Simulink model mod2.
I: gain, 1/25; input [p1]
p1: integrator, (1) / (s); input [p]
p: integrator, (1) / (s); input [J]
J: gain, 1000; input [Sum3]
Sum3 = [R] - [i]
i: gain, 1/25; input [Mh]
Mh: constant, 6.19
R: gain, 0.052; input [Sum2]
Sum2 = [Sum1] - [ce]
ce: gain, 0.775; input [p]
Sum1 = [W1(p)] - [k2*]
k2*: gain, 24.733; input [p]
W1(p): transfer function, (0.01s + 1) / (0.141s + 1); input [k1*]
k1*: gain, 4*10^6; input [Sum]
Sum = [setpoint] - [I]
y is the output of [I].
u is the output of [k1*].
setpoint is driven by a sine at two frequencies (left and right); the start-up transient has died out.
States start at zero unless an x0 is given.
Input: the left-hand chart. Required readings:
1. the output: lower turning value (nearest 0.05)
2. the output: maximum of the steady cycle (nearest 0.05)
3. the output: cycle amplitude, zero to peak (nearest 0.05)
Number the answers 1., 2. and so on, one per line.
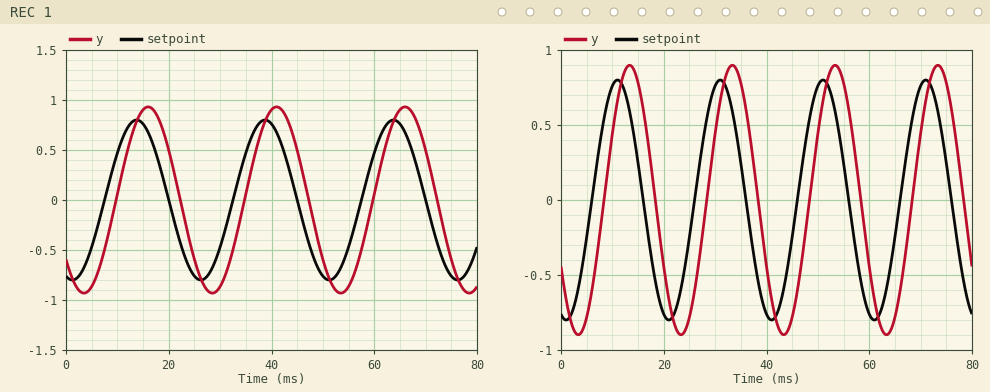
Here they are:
1. -0.95
2. 0.95
3. 0.95
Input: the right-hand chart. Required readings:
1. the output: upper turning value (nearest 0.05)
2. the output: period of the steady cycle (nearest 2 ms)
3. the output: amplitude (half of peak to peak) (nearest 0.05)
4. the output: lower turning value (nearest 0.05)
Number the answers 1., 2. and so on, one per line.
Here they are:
1. 0.90
2. 20 ms
3. 0.90
4. -0.90
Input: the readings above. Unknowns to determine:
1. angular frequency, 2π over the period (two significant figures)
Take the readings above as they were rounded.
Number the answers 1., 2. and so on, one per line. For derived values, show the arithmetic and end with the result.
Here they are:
1. 2π / 20 = 0.31 rad/ms
